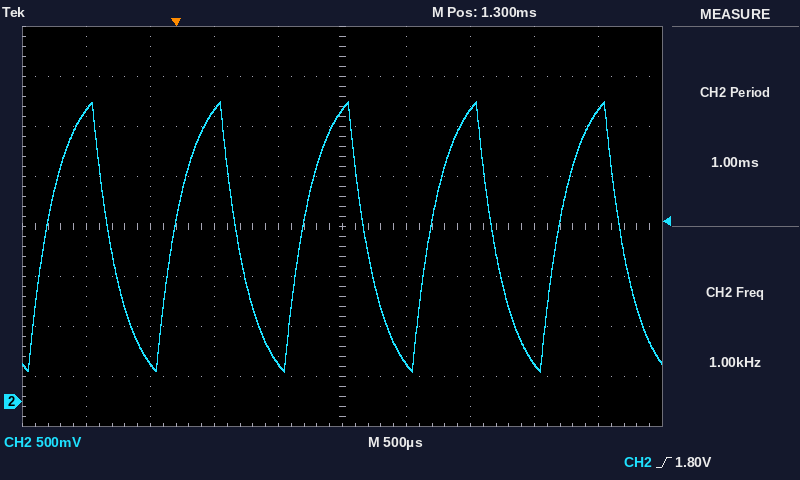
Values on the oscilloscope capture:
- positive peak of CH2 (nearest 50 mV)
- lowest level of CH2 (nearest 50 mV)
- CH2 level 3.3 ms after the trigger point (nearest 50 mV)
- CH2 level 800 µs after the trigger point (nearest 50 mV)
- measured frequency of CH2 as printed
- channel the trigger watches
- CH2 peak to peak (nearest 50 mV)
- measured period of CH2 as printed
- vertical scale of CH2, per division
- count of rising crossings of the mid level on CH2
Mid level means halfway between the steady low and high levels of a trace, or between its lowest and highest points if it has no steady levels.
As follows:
3.00 V
300 mV
2.90 V
400 mV
1.00 kHz
CH2
2.70 V
1.00 ms
500 mV
5
